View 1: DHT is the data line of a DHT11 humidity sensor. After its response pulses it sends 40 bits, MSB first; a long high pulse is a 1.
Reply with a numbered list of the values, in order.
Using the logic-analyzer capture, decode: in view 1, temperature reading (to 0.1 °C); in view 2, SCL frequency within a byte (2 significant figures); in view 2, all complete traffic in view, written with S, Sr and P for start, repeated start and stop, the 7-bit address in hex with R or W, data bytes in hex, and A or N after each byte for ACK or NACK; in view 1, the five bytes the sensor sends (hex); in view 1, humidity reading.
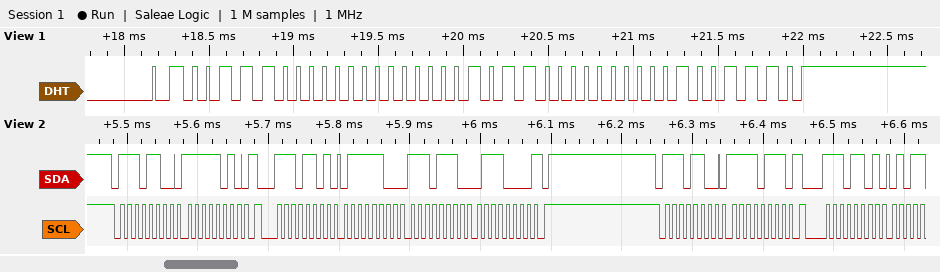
1. 22.0 °C
2. 100 kHz
3. S 76W A FA A Sr 76R A 7C A EE A 70 N P S 76W A F7 A Sr 76R A
4. 38 00 16 00 4E
5. 56 %
